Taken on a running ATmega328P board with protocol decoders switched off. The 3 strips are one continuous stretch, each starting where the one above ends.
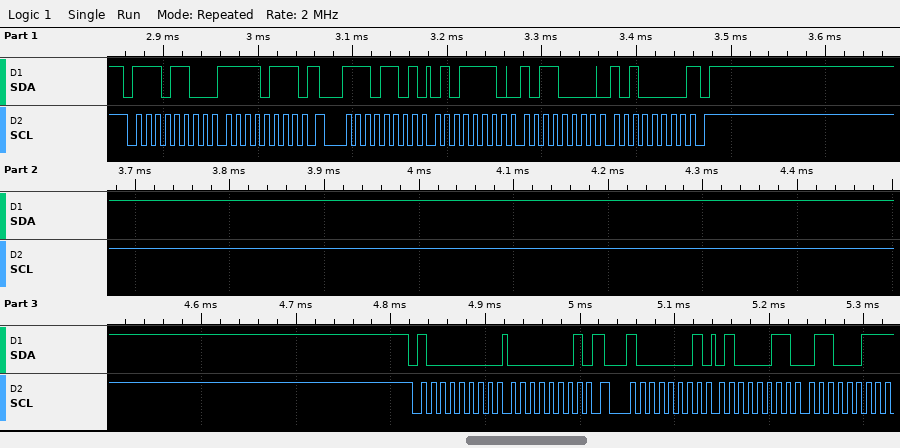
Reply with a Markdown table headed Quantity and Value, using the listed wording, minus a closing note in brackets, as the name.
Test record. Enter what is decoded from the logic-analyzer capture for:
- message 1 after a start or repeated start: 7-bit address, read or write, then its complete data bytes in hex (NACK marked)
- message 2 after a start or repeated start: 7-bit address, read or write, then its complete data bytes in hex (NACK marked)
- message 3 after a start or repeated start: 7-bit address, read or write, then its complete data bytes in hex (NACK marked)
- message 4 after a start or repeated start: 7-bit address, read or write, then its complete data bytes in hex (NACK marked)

| Quantity | Value |
|---|---|
| message 1 after a start or repeated start: 7-bit address, read or write, then its complete data bytes in hex | 0x76 write: F7 |
| message 2 after a start or repeated start: 7-bit address, read or write, then its complete data bytes in hex | 0x76 read: 5E B0 A0 NACK |
| message 3 after a start or repeated start: 7-bit address, read or write, then its complete data bytes in hex | 0x40 write: 01 |
| message 4 after a start or repeated start: 7-bit address, read or write, then its complete data bytes in hex | 0x40 read: 43 63 NACK |
